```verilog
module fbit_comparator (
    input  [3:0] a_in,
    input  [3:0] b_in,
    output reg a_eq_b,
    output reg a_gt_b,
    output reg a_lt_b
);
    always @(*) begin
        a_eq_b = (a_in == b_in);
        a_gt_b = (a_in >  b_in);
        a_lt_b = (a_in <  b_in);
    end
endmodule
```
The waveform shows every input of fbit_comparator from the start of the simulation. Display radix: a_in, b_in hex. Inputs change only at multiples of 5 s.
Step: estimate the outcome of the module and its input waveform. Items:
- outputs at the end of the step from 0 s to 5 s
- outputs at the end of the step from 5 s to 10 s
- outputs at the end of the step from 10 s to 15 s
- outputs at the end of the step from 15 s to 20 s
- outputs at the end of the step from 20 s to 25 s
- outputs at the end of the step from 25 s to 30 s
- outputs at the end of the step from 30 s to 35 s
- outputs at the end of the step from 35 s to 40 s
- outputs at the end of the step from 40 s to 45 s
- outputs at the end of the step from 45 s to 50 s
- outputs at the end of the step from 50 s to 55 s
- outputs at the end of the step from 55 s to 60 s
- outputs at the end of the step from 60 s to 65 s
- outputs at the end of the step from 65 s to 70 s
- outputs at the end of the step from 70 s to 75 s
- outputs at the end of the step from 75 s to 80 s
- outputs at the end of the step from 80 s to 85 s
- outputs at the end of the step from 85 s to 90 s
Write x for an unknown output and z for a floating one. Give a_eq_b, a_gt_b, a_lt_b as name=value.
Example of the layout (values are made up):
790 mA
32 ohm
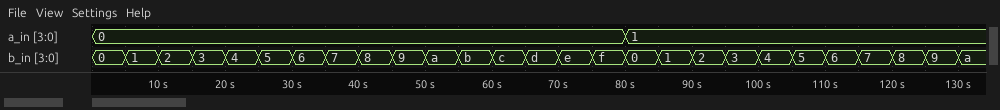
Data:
a_eq_b=1, a_gt_b=0, a_lt_b=0
a_eq_b=0, a_gt_b=0, a_lt_b=1
a_eq_b=0, a_gt_b=0, a_lt_b=1
a_eq_b=0, a_gt_b=0, a_lt_b=1
a_eq_b=0, a_gt_b=0, a_lt_b=1
a_eq_b=0, a_gt_b=0, a_lt_b=1
a_eq_b=0, a_gt_b=0, a_lt_b=1
a_eq_b=0, a_gt_b=0, a_lt_b=1
a_eq_b=0, a_gt_b=0, a_lt_b=1
a_eq_b=0, a_gt_b=0, a_lt_b=1
a_eq_b=0, a_gt_b=0, a_lt_b=1
a_eq_b=0, a_gt_b=0, a_lt_b=1
a_eq_b=0, a_gt_b=0, a_lt_b=1
a_eq_b=0, a_gt_b=0, a_lt_b=1
a_eq_b=0, a_gt_b=0, a_lt_b=1
a_eq_b=0, a_gt_b=0, a_lt_b=1
a_eq_b=0, a_gt_b=1, a_lt_b=0
a_eq_b=1, a_gt_b=0, a_lt_b=0
